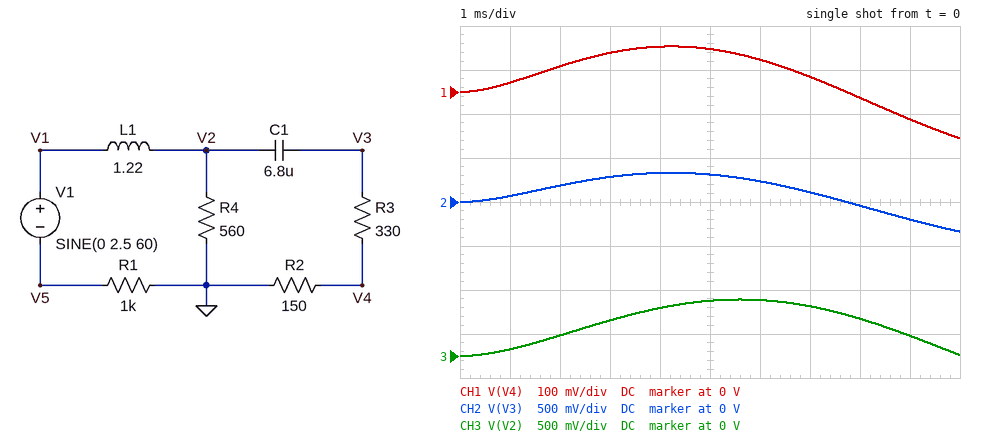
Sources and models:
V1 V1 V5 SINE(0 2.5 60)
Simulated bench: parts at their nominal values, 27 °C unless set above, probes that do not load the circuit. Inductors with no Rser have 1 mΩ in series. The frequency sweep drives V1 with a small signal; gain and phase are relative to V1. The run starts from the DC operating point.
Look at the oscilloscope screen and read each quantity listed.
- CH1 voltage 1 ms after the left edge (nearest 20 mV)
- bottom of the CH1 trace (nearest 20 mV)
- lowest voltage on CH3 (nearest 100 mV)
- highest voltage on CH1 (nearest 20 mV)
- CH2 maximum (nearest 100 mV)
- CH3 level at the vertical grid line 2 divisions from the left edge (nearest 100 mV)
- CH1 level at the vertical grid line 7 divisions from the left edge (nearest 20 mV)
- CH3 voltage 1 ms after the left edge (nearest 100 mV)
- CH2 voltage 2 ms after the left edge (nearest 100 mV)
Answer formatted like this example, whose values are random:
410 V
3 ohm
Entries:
20 mV
-100 mV
0 V
100 mV
300 mV
200 mV
40 mV
100 mV
200 mV
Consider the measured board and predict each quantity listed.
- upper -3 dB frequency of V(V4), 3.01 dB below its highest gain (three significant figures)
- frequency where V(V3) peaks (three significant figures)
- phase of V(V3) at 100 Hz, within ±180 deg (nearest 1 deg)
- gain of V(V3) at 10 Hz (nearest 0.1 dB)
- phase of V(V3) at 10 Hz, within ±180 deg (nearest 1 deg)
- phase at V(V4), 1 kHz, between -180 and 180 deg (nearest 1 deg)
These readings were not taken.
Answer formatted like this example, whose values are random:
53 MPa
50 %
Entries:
209 Hz
67.7 Hz
-16 deg
-23.2 dB
67 deg
-79 deg
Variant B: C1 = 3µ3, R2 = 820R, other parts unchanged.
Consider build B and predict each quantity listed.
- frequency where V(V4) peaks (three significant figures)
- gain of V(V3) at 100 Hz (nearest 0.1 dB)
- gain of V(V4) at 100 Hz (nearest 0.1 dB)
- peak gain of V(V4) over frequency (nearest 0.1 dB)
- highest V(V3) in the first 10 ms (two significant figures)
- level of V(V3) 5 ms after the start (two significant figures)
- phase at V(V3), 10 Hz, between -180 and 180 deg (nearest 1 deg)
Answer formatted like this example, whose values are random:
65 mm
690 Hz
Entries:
75.8 Hz
-12.7 dB
-15.6 dB
-15.5 dB
420 mV
390 mV
70 deg
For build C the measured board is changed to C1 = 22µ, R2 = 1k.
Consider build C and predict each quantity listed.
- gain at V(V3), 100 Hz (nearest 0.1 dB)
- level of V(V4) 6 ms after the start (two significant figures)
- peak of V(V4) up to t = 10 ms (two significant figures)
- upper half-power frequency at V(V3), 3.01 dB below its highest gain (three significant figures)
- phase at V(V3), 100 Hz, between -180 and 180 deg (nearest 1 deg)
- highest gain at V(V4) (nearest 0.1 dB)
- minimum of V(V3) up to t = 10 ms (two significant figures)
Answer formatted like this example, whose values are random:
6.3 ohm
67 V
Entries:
-12.1 dB
420 mV
470 mV
190 Hz
-26 deg
-13.6 dB
-290 mV
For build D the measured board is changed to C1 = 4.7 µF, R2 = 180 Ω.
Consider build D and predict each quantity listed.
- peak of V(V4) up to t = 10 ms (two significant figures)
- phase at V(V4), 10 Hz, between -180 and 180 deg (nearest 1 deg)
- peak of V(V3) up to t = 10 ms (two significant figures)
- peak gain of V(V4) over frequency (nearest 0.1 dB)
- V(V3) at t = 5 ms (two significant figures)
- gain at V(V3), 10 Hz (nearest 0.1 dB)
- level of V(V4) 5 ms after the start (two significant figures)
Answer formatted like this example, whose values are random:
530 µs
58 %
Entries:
110 mV
73 deg
300 mV
-24.1 dB
270 mV
-25.6 dB
96 mV
